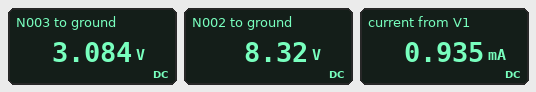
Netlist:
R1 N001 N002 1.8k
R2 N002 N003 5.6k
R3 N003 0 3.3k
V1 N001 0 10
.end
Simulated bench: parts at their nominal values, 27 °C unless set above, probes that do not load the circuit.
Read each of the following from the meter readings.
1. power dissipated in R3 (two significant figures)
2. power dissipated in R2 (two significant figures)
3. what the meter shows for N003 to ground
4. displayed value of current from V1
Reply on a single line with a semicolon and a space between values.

2.9 mW; 4.9 mW; 3.084 V; 0.935 mA
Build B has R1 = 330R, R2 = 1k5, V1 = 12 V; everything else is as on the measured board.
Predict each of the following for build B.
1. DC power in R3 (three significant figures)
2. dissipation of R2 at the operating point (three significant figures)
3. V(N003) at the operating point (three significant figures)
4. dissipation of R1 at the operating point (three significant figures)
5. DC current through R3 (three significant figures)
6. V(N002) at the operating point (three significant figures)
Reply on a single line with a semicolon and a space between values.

18.1 mW; 8.21 mW; 7.72 V; 1.81 mW; 2.34 mA; 11.2 V
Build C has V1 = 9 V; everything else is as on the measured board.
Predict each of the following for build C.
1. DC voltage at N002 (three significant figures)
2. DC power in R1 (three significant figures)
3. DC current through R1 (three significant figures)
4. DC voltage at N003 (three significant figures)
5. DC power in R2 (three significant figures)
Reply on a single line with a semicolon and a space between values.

7.49 V; 1.27 mW; 841 µA; 2.78 V; 3.96 mW
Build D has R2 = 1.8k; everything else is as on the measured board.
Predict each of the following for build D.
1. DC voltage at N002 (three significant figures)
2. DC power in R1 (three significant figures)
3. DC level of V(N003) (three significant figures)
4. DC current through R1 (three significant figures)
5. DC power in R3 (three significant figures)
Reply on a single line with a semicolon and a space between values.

7.39 V; 3.78 mW; 4.78 V; 1.45 mA; 6.93 mW
